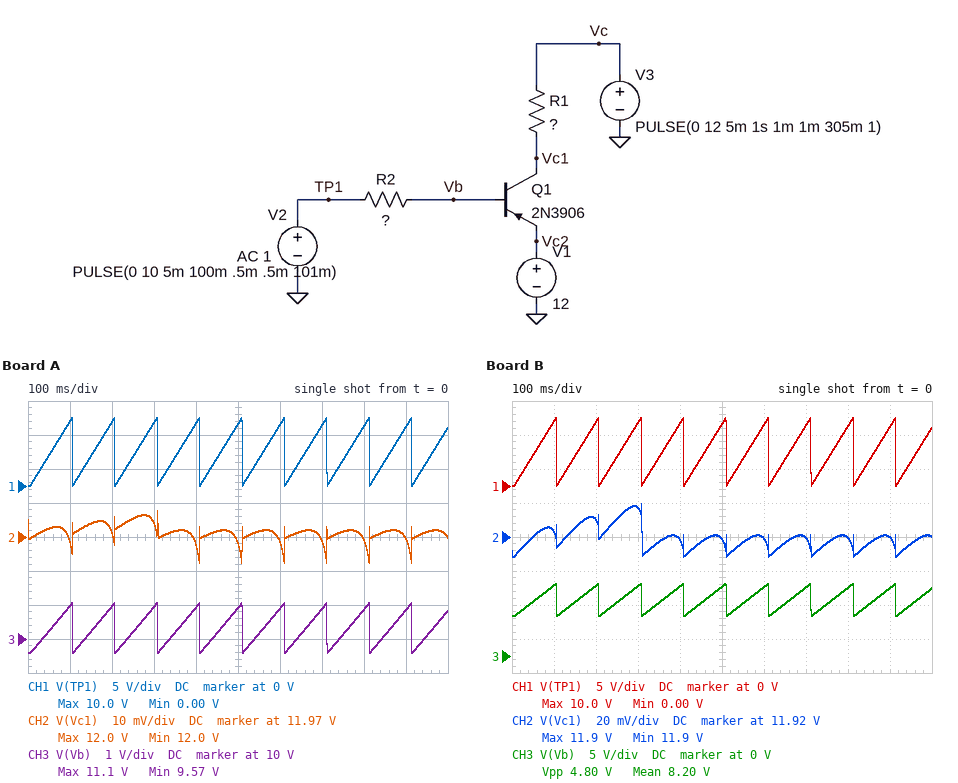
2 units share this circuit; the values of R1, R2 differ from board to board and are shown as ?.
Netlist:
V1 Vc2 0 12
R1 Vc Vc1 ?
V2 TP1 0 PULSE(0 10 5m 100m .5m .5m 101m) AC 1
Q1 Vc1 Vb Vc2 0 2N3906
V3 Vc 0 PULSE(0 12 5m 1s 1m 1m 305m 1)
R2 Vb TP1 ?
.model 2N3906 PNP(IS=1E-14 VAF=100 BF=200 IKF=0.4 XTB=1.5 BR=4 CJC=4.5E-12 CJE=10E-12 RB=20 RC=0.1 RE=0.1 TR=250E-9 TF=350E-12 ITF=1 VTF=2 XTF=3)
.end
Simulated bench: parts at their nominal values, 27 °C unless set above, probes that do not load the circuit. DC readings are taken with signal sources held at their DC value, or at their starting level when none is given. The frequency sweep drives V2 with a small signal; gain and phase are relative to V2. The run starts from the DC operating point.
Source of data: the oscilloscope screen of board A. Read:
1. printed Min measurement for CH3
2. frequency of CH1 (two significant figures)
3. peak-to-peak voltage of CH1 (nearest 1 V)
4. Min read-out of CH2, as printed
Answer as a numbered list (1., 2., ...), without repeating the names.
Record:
1. 9.57 V
2. 9.9 Hz
3. 10 V
4. 12.0 V
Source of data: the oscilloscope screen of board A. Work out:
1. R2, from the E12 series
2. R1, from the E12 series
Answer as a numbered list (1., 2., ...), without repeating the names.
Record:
1. 120 Ω
2. 270 Ω
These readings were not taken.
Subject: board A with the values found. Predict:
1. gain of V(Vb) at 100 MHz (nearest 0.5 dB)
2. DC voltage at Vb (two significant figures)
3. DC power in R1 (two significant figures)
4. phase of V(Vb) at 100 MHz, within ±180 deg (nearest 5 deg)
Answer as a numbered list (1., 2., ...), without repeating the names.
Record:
1. -17.0 dB
2. 9.6 V
3. 530 mW
4. 0 deg
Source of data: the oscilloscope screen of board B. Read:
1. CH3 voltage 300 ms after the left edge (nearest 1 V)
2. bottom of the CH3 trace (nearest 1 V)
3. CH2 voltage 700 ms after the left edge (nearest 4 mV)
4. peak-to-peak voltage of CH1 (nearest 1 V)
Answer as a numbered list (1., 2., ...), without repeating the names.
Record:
1. 10 V
2. 6 V
3. 11.920 V
4. 10 V
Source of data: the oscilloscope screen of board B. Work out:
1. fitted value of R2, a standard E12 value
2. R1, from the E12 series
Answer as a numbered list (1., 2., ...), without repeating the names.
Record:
1. 22 Ω
2. 56 Ω
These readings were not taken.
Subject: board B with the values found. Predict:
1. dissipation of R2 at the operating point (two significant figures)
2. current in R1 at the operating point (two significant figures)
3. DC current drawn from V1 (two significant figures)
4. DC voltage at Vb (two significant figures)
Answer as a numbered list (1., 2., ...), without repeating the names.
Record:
1. 1.5 W
2. 210 mA
3. 480 mA
4. 5.8 V
